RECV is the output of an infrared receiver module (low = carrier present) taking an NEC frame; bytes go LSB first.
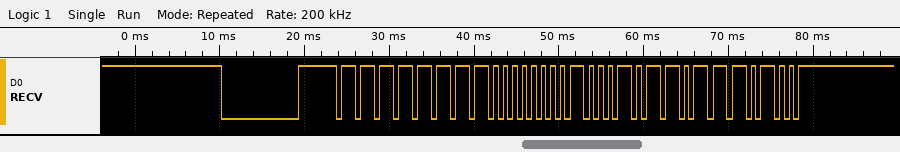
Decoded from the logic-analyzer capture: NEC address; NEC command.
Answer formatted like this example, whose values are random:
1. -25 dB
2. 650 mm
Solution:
1. 0xFF
2. 0xD1
